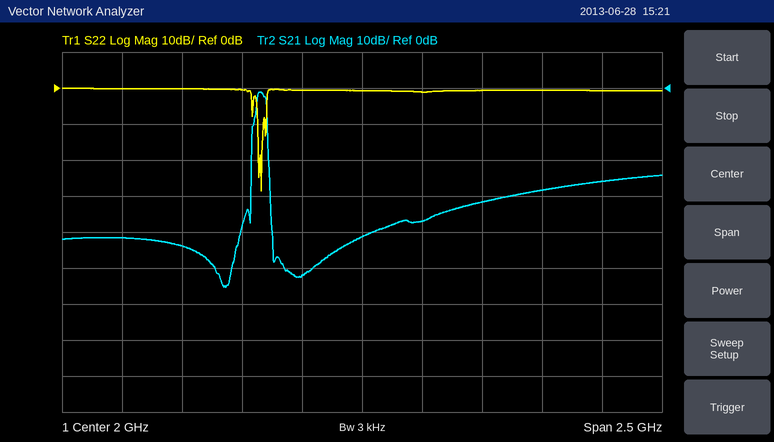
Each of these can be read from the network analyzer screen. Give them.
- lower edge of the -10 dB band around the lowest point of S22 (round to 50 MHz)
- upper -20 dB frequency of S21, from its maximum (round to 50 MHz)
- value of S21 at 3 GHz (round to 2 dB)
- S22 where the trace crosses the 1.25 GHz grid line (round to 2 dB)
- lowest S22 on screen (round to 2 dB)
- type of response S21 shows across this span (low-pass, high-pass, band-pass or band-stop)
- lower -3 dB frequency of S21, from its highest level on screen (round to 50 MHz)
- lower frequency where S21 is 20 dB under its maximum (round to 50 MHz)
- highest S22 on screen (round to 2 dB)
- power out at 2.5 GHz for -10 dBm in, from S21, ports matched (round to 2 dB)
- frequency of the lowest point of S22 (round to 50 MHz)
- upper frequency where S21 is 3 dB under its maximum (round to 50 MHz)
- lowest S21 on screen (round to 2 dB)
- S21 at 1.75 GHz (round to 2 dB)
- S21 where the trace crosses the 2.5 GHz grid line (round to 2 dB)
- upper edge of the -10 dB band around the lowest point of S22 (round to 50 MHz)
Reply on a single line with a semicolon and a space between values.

1.55 GHz; 1.60 GHz; -26 dB; 0 dB; -28 dB; band-pass; 1.55 GHz; 1.55 GHz; 0 dB; -42 dBm; 1.60 GHz; 1.60 GHz; -56 dB; -52 dB; -32 dB; 1.60 GHz
